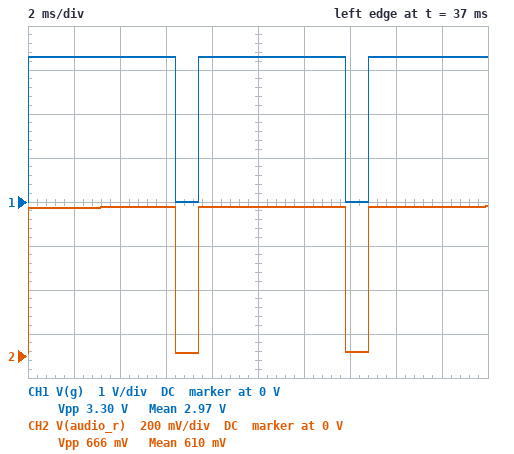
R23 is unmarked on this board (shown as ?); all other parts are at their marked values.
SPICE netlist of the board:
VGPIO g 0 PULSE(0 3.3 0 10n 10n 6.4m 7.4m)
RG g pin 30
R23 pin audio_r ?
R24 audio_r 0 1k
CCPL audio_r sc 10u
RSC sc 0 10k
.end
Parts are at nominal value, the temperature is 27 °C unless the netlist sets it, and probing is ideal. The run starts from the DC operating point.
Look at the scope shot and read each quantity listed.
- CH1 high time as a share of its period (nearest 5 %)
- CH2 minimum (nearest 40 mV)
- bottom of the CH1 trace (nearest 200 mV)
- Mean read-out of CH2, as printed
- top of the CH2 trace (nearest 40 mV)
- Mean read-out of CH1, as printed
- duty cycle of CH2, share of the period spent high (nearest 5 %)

85 %
0 V
0 V
610 mV
680 mV
2.97 V
85 %
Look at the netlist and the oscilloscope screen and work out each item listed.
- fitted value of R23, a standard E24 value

3.6 kΩ
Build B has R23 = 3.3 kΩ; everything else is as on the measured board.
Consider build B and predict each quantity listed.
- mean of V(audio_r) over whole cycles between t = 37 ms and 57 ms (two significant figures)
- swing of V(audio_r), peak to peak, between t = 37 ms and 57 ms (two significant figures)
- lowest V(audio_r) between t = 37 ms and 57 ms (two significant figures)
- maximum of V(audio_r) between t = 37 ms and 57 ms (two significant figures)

630 mV
710 mV
14 mV
730 mV
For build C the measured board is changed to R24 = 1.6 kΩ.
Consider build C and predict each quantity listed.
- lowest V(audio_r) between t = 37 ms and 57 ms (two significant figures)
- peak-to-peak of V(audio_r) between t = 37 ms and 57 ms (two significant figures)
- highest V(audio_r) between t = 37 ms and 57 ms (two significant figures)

25 mV
920 mV
940 mV
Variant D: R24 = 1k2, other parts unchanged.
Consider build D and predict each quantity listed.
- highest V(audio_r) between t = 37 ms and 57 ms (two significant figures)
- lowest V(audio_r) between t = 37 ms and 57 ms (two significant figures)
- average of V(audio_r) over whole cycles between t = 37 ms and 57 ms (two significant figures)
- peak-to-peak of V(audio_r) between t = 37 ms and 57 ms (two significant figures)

780 mV
17 mV
670 mV
760 mV
